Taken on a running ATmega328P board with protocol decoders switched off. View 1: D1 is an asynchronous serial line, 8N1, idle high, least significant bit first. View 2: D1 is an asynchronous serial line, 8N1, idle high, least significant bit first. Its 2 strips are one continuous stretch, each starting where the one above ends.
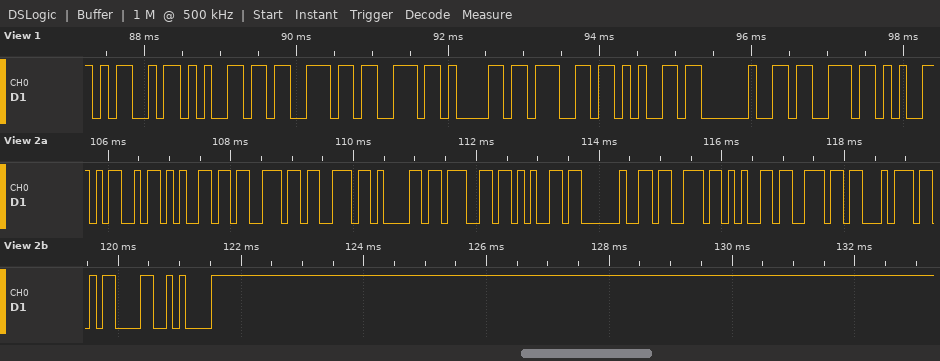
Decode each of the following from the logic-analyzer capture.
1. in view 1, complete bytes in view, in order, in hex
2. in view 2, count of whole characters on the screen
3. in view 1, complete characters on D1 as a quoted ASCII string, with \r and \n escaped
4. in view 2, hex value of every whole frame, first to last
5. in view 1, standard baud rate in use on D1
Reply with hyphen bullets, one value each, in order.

- 4D 65 73 73 61 67 65 20 73
- 14
- "Message s"
- 4D 65 73 73 61 67 65 20 73 65 6E 74 0D 0A
- 9600 baud
